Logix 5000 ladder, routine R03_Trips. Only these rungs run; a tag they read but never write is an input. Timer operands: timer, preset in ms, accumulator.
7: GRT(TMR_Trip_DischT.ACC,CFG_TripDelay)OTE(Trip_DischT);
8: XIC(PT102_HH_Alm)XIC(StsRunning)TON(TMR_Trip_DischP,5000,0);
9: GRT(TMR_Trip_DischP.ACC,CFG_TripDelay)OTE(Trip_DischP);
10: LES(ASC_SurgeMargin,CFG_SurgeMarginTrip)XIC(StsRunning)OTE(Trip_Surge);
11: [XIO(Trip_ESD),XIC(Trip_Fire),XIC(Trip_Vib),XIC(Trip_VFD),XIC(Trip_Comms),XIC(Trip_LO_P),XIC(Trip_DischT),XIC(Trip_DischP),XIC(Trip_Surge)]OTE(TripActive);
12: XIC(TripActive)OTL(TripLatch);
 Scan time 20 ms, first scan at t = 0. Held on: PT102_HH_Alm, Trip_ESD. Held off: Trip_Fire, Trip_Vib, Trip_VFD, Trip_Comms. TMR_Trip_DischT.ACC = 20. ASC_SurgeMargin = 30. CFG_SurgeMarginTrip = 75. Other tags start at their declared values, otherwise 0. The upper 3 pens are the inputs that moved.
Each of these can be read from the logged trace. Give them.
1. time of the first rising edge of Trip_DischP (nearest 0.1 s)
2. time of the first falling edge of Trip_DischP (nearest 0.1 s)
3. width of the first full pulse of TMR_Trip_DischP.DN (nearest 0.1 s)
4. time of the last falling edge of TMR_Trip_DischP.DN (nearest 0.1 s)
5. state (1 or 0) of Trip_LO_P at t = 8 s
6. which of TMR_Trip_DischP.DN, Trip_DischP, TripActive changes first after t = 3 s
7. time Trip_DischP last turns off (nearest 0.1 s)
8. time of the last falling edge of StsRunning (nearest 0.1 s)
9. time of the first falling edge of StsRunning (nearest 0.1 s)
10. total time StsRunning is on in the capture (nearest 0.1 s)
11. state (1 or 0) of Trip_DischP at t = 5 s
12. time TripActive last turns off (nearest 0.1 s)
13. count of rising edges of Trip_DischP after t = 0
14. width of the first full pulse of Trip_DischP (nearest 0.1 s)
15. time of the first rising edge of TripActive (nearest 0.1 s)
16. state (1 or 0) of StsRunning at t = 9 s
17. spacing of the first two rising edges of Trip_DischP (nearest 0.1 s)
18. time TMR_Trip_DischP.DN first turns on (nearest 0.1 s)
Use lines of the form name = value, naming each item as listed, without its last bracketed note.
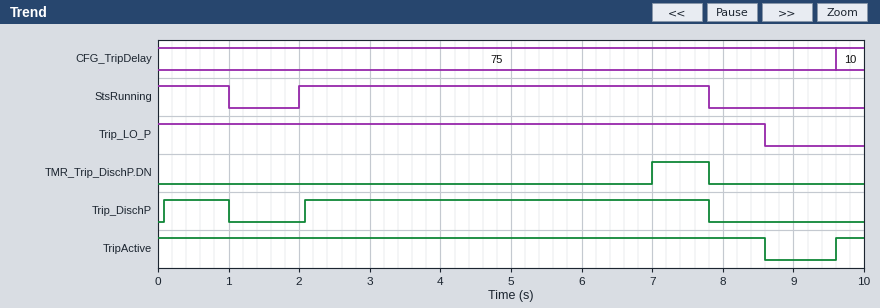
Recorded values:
time of the first rising edge of Trip_DischP = 0.1 s
time of the first falling edge of Trip_DischP = 1.0 s
width of the first full pulse of TMR_Trip_DischP.DN = 0.8 s
time of the last falling edge of TMR_Trip_DischP.DN = 7.8 s
state (1 or 0) of Trip_LO_P at t = 8 s = 1
which of TMR_Trip_DischP.DN, Trip_DischP, TripActive changes first after t = 3 s = TMR_Trip_DischP.DN
time Trip_DischP last turns off = 7.8 s
time of the last falling edge of StsRunning = 7.8 s
time of the first falling edge of StsRunning = 1.0 s
total time StsRunning is on in the capture = 6.8 s
state (1 or 0) of Trip_DischP at t = 5 s = 1
time TripActive last turns off = 8.6 s
count of rising edges of Trip_DischP after t = 0 = 2
width of the first full pulse of Trip_DischP = 0.9 s
time of the first rising edge of TripActive = 9.6 s
state (1 or 0) of StsRunning at t = 9 s = 0
spacing of the first two rising edges of Trip_DischP = 2.0 s
time TMR_Trip_DischP.DN first turns on = 7.0 s
